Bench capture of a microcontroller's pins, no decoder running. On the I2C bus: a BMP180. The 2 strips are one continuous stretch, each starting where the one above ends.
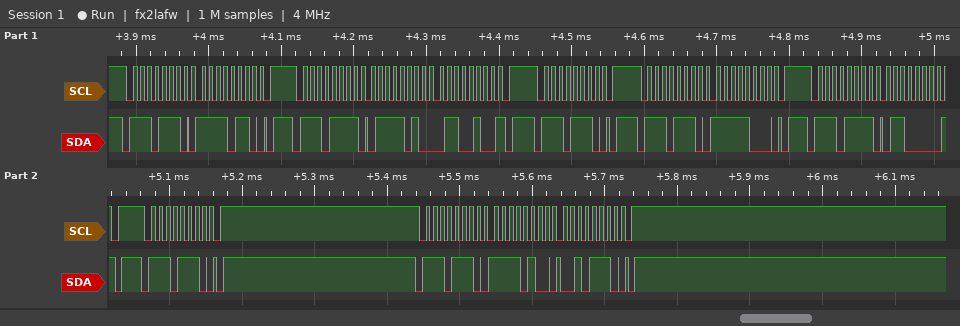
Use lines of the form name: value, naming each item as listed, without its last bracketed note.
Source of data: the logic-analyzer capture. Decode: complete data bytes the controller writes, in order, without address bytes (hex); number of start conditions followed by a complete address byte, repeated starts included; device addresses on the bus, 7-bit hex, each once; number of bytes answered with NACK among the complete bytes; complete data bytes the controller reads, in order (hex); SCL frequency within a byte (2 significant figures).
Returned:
complete data bytes the controller writes, in order, without address bytes: F6 F8 F4 2E
number of start conditions followed by a complete address byte, repeated starts included: 7
device addresses on the bus, 7-bit hex, each once: 0x77
number of bytes answered with NACK among the complete bytes: 2
complete data bytes the controller reads, in order: 7A 64 60
SCL frequency within a byte: 100 kHz
